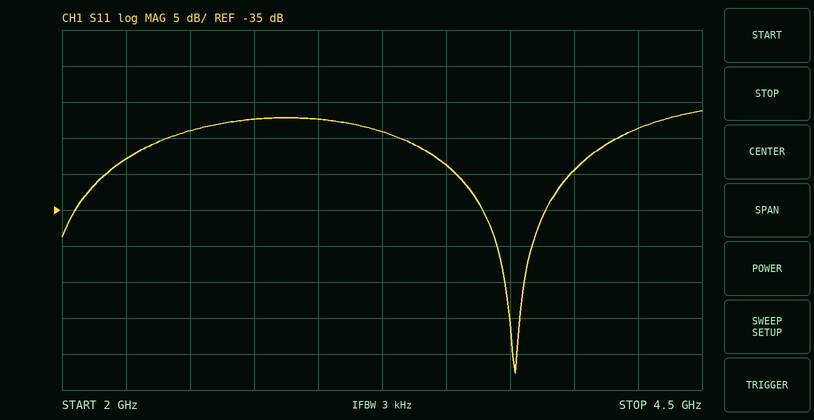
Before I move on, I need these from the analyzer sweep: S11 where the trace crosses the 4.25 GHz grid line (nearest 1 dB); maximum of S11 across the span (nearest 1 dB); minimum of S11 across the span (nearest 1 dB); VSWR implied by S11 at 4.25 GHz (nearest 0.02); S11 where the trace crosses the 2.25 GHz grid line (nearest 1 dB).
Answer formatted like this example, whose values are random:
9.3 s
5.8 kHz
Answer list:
-24 dB
-21 dB
-58 dB
1.14
-28 dB
